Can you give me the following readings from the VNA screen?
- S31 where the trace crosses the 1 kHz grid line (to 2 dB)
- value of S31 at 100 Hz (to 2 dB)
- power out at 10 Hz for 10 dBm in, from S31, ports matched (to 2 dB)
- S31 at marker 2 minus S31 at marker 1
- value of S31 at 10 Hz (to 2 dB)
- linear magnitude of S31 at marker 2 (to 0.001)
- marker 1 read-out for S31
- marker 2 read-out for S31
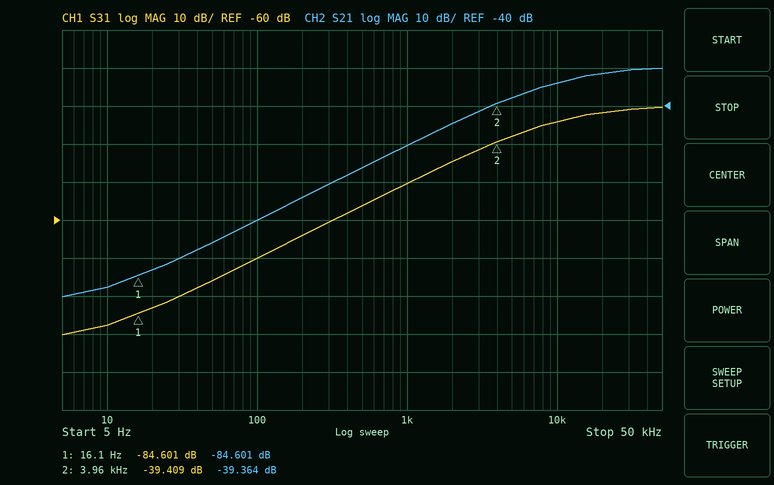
-50 dB
-70 dB
-78 dBm
45.192 dB
-88 dB
0.011
-84.601 dB
-39.409 dB
